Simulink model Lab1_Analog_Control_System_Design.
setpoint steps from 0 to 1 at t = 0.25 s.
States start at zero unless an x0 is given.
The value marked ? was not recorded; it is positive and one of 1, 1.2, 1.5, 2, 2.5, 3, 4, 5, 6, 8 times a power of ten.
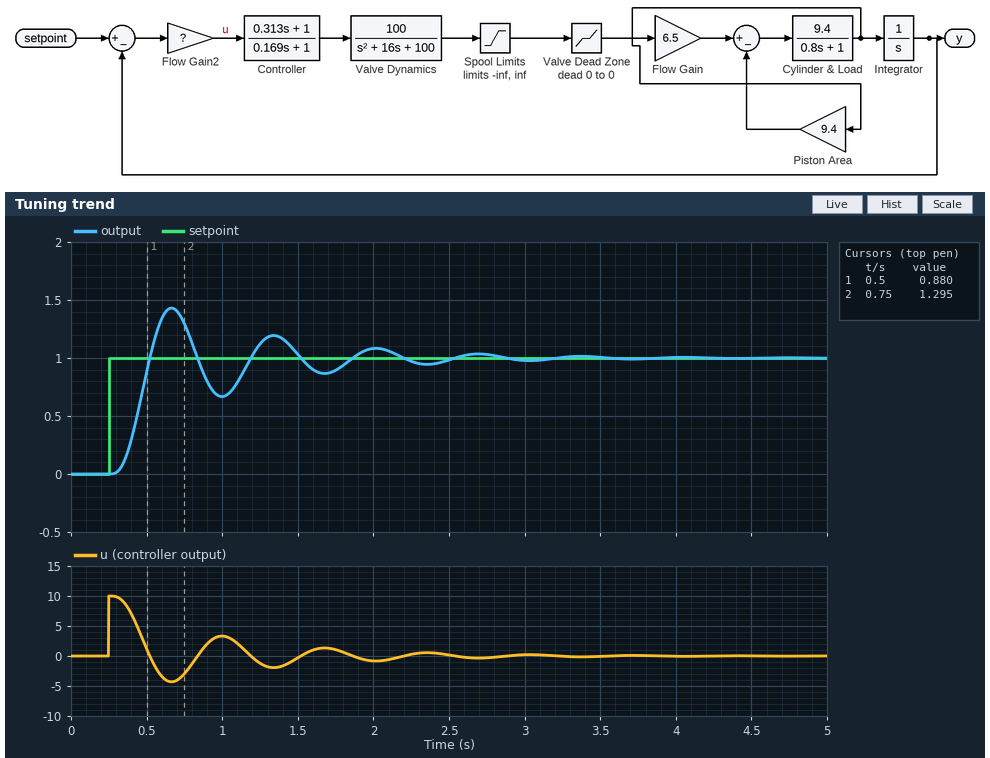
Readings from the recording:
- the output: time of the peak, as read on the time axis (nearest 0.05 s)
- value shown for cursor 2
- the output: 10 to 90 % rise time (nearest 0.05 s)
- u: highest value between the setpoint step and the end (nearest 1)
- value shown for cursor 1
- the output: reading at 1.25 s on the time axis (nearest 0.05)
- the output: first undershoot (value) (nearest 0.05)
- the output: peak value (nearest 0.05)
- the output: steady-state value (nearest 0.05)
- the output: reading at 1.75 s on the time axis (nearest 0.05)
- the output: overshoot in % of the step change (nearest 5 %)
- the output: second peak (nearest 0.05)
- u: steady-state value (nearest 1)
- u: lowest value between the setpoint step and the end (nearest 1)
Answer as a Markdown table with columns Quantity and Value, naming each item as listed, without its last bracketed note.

| Quantity | Value |
|---|---|
| the output: time of the peak, as read on the time axis | 0.65 s |
| value shown for cursor 2 | 1.295 |
| the output: 10 to 90 % rise time | 0.15 s |
| u: highest value between the setpoint step and the end | 10 |
| value shown for cursor 1 | 0.880 |
| the output: reading at 1.25 s on the time axis | 1.10 |
| the output: first undershoot (value) | 0.65 |
| the output: peak value | 1.45 |
| the output: steady-state value | 1.00 |
| the output: reading at 1.75 s on the time axis | 0.90 |
| the output: overshoot in % of the step change | 45 % |
| the output: second peak | 1.20 |
| u: steady-state value | 0 |
| u: lowest value between the setpoint step and the end | -4 |
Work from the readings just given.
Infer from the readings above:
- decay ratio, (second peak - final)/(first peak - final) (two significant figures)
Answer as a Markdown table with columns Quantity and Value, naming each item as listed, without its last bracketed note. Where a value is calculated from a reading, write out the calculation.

| Quantity | Value |
|---|---|
| decay ratio, (second peak - final)/(first peak - final) | (1.2 - 1) / (1.45 - 1) = 0.44 |
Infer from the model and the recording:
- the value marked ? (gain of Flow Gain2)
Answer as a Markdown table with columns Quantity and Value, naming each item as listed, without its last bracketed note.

| Quantity | Value |
|---|---|
| the value marked ? | 10 |
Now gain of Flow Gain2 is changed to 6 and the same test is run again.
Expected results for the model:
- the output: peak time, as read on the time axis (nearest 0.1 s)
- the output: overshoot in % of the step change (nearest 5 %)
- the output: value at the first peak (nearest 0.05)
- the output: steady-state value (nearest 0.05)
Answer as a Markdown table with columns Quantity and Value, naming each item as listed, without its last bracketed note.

| Quantity | Value |
|---|---|
| the output: peak time, as read on the time axis | 0.8 s |
| the output: overshoot in % of the step change | 15 % |
| the output: value at the first peak | 1.15 |
| the output: steady-state value | 1.00 |
